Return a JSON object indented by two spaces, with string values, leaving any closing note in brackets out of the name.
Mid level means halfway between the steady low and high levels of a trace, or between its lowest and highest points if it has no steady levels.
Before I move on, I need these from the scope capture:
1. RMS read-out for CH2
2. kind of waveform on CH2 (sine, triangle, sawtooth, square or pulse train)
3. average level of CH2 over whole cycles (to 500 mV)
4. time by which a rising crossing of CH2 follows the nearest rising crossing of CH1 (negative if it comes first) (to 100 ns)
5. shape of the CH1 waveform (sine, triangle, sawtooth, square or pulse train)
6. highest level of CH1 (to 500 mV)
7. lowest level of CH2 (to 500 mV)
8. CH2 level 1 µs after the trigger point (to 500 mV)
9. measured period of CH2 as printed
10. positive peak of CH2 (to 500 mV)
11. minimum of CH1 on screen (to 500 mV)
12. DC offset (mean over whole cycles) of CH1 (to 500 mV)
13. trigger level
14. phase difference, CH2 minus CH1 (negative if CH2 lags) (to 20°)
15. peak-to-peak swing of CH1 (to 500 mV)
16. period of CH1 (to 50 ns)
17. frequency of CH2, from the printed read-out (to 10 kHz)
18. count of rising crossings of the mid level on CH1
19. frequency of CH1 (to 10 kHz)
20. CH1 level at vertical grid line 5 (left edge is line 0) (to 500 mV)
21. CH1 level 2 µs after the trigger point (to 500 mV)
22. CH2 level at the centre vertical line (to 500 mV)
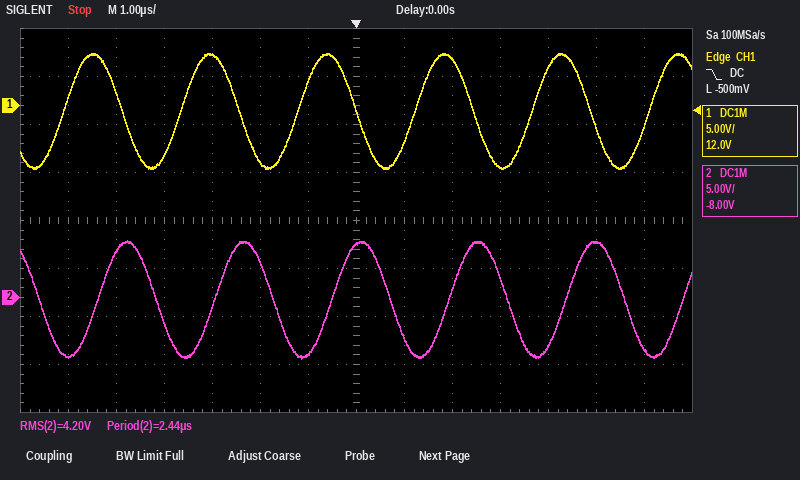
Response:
{
  "RMS read-out for CH2": "4.20 V",
  "kind of waveform on CH2": "sine",
  "average level of CH2 over whole cycles": "0.0 V",
  "time by which a rising crossing of CH2 follows the nearest rising crossing of CH1 (negative if it comes first)": "+700 ns",
  "shape of the CH1 waveform": "sine",
  "highest level of CH1": "5.5 V",
  "lowest level of CH2": "-6.5 V",
  "CH2 level 1 µs after the trigger point": "-4.0 V",
  "measured period of CH2 as printed": "2.44 µs",
  "positive peak of CH2": "6.0 V",
  "minimum of CH1 on screen": "-6.5 V",
  "DC offset (mean over whole cycles) of CH1": "-500 mV",
  "trigger level": "-500 mV",
  "phase difference, CH2 minus CH1 (negative if CH2 lags)": "-100°",
  "peak-to-peak swing of CH1": "12.0 V",
  "period of CH1": "2.45 µs",
  "frequency of CH2, from the printed read-out": "410 kHz",
  "count of rising crossings of the mid level on CH1": "6",
  "frequency of CH1": "410 kHz",
  "CH1 level at vertical grid line 5 (left edge is line 0)": "-6.0 V",
  "CH1 level 2 µs after the trigger point": "5.0 V",
  "CH2 level at the centre vertical line": "5.5 V"
}
